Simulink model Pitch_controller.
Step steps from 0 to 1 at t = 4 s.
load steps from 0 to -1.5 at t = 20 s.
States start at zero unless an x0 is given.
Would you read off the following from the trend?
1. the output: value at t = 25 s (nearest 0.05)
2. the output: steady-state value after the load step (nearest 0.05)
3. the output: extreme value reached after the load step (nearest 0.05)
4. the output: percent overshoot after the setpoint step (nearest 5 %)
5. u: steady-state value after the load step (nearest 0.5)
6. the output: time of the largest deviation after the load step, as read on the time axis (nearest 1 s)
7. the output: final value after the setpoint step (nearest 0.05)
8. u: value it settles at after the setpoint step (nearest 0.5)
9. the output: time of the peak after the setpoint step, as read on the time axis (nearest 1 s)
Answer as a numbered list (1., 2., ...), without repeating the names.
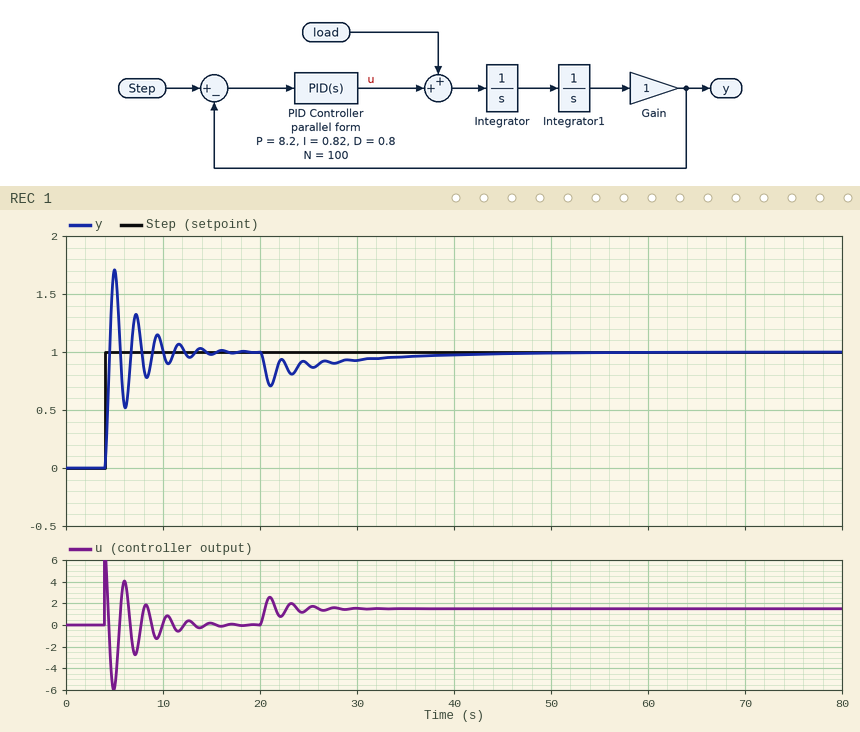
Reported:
1. 0.90
2. 1.00
3. 0.70
4. 70 %
5. 1.5
6. 21 s
7. 1.00
8. 0.0
9. 5 s
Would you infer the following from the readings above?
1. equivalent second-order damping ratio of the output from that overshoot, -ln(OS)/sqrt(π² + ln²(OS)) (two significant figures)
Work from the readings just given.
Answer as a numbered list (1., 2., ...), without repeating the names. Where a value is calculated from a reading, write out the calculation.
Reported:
1. ln(0.7) = -0.357; 0.357 / sqrt(9.870 + 0.127) = 0.11
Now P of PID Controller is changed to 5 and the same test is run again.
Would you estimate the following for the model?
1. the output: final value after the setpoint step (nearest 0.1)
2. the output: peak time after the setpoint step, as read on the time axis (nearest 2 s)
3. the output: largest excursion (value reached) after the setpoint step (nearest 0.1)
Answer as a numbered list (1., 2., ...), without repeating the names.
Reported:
1. 1.0
2. 6 s
3. 1.7
